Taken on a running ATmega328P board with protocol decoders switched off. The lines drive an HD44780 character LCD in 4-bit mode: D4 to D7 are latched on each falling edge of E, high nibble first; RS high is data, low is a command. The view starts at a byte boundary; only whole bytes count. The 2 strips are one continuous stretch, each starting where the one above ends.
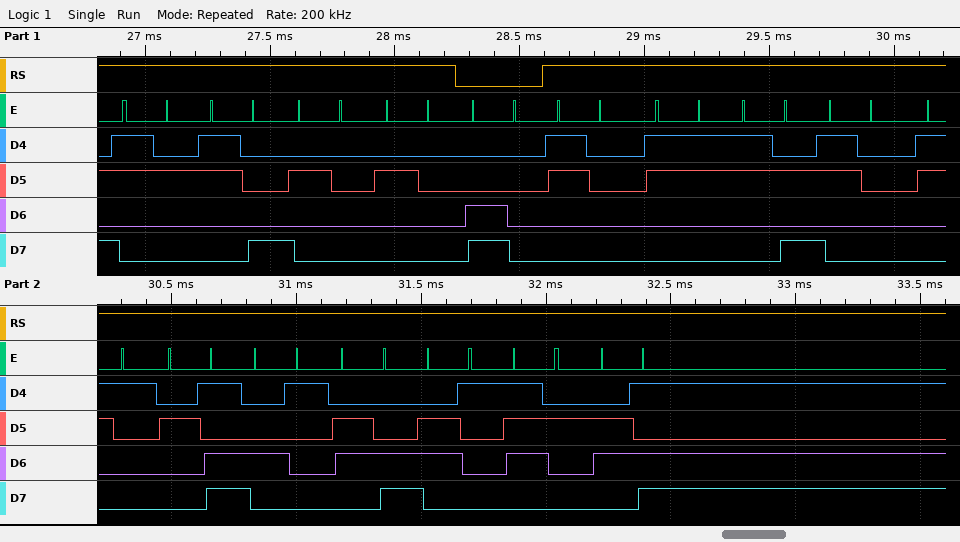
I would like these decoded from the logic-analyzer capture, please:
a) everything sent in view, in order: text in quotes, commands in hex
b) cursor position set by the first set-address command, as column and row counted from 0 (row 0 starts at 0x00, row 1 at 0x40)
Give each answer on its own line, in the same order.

"28  " 0xC0 "03:01-Alarm"
column 0, row 1
